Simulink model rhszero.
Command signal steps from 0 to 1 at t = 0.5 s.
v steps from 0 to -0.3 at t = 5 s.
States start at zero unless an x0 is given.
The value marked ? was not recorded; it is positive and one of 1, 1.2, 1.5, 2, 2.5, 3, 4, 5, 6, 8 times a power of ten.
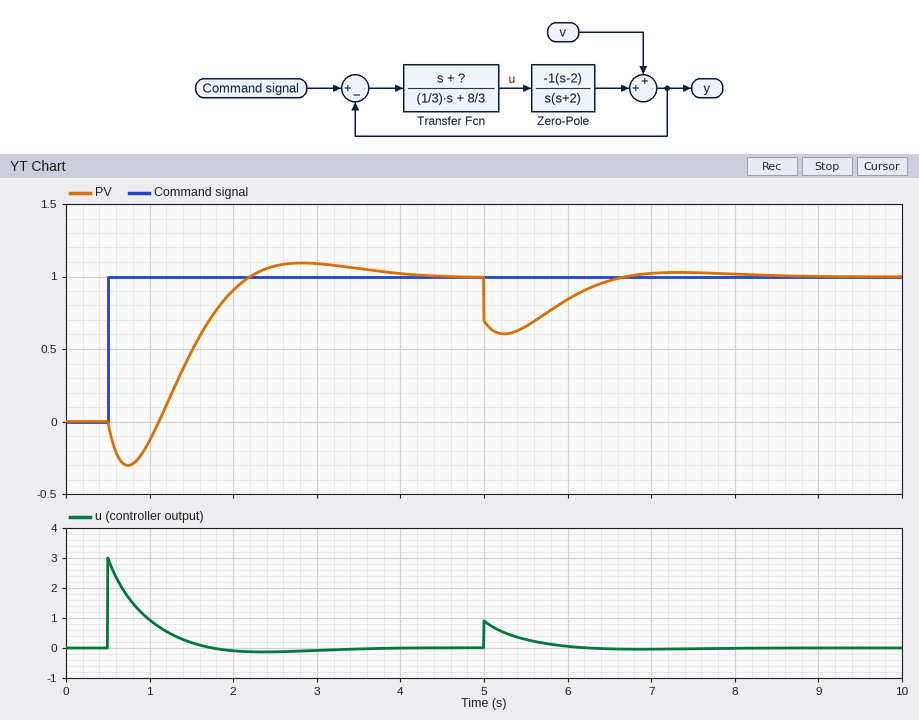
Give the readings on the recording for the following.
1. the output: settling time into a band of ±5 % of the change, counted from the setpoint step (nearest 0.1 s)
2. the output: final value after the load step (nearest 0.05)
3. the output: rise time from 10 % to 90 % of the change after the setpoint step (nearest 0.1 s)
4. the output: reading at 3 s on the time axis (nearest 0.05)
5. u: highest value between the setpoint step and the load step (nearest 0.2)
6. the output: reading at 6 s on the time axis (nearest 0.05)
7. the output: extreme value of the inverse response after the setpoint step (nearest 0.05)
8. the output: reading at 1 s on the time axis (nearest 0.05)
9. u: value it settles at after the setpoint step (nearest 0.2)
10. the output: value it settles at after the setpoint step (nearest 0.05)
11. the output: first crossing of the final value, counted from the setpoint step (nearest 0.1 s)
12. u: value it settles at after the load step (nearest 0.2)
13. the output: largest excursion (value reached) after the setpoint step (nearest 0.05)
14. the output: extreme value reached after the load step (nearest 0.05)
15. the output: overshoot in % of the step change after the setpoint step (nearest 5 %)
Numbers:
3.1 s
1.00
0.8 s
1.10
3.0
0.85
-0.30
-0.15
0.0
1.00
1.7 s
0.0
1.10
0.60
10 %
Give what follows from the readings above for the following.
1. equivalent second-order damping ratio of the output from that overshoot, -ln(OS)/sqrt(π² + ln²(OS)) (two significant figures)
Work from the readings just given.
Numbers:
0.59
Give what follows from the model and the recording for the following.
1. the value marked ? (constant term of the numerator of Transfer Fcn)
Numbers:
2.5
